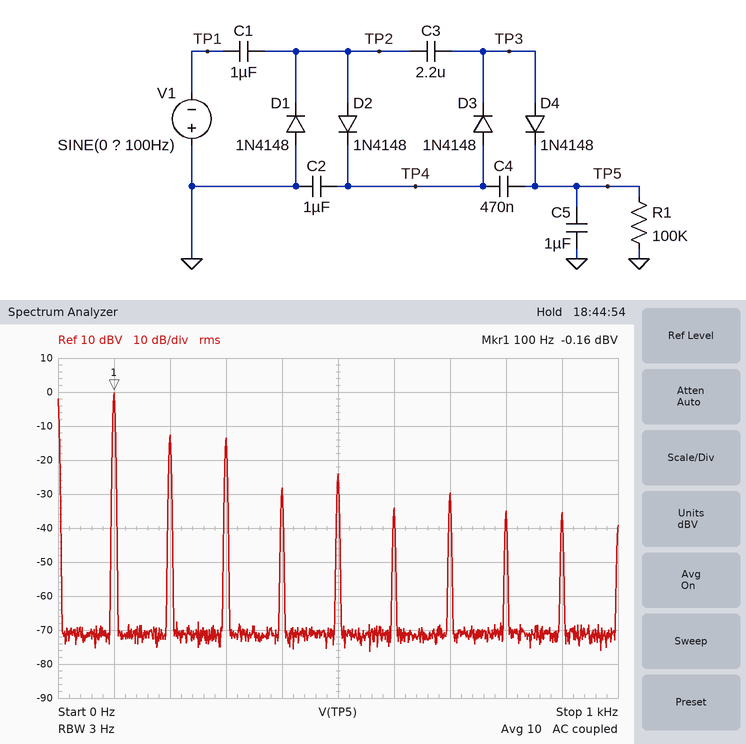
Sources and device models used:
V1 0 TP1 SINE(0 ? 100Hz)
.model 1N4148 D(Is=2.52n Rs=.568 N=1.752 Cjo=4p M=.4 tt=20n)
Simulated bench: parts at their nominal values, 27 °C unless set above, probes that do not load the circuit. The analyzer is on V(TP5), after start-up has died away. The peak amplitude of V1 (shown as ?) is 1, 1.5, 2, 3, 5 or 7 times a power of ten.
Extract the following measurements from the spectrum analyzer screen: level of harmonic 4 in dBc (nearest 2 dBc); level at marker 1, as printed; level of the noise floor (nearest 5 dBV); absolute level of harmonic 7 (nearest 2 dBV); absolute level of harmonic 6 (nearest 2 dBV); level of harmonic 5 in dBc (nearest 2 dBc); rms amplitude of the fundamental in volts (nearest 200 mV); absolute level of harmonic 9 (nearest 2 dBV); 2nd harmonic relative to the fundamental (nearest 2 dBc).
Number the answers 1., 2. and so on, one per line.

1. -28 dBc
2. -0.16 dBV
3. -70 dBV
4. -30 dBV
5. -34 dBV
6. -24 dBc
7. 1.0 V
8. -36 dBV
9. -12 dBc
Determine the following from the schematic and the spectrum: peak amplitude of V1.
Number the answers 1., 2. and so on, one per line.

1. 15 V
